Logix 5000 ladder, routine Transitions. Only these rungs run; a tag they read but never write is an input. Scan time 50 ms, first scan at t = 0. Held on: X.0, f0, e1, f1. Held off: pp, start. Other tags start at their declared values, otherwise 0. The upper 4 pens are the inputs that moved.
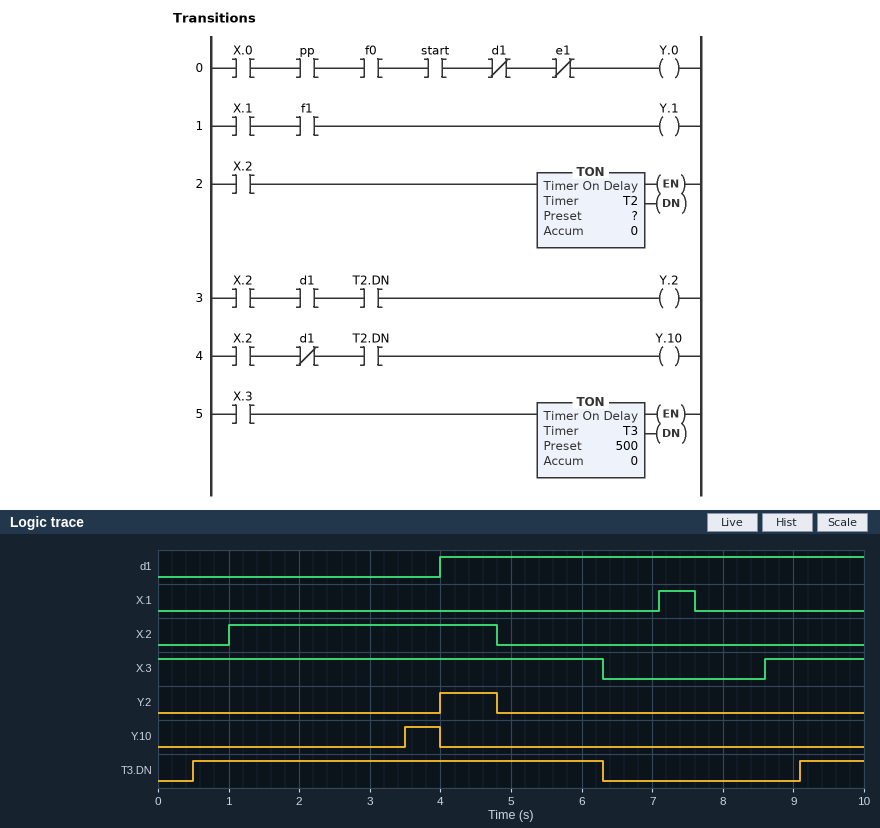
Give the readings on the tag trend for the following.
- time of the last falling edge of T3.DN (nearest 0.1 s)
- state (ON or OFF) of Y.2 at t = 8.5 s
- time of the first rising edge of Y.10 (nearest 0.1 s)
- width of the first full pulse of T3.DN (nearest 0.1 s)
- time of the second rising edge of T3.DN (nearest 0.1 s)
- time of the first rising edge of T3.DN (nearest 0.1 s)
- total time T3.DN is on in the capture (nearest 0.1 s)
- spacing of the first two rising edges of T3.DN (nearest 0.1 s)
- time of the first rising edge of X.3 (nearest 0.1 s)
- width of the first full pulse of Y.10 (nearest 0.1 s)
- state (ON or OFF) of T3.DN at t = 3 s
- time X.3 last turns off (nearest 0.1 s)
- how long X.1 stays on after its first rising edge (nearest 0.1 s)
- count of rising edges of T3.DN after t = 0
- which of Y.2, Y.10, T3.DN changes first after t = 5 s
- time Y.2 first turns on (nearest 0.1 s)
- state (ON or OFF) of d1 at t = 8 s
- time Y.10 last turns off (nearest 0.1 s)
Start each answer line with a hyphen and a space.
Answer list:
- 6.3 s
- OFF
- 3.5 s
- 5.8 s
- 9.1 s
- 0.5 s
- 6.7 s
- 8.6 s
- 8.6 s
- 0.5 s
- ON
- 6.3 s
- 0.5 s
- 2
- T3.DN
- 4.0 s
- ON
- 4.0 s
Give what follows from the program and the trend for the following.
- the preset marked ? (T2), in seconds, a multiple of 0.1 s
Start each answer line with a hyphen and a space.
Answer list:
- 2.5 s
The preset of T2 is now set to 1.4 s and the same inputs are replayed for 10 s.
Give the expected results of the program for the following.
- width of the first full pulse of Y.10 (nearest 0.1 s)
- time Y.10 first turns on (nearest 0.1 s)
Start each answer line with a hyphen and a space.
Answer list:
- 1.6 s
- 2.4 s
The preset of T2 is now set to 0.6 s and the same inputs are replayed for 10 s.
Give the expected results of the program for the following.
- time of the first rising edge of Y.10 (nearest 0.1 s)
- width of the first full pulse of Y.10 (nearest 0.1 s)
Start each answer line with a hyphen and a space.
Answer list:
- 1.6 s
- 2.4 s
